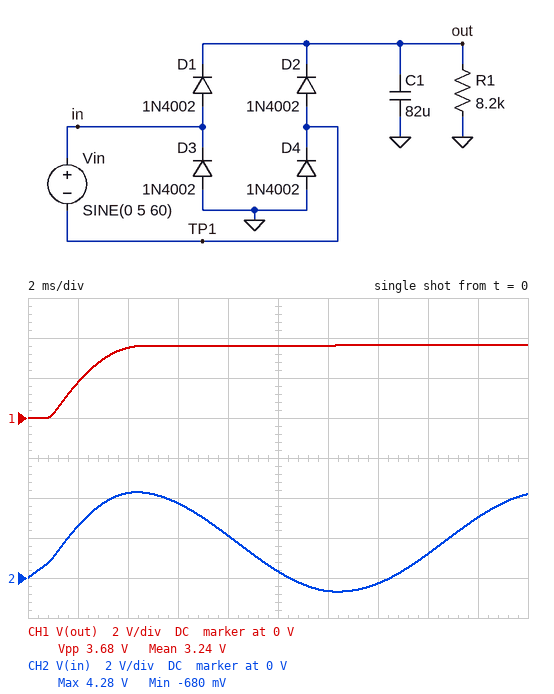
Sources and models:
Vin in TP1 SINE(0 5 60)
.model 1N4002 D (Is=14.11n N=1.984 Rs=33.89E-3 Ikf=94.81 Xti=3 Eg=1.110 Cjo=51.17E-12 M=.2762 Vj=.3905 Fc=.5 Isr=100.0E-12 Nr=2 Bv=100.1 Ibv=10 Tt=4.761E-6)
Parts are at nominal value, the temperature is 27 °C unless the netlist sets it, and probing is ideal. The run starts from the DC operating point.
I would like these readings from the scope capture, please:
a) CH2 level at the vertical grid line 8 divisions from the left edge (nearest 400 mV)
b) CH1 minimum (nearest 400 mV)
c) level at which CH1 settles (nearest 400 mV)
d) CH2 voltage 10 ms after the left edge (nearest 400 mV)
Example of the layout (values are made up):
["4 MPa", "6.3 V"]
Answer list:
["1.2 V", "0 V", "3.6 V", "400 mV"]
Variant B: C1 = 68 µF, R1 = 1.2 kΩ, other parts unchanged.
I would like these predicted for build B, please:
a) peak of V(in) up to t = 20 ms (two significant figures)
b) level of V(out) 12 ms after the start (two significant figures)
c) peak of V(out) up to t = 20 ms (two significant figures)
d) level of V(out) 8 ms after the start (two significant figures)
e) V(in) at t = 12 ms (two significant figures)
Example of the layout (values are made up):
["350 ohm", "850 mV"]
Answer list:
["4.3 V", "3.4 V", "3.6 V", "3.5 V", "-740 mV"]
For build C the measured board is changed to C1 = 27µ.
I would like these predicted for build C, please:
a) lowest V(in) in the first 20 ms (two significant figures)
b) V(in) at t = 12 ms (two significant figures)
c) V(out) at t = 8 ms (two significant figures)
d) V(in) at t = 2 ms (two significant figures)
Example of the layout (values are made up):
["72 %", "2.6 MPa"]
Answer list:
["-650 mV", "-630 mV", "3.7 V", "2.7 V"]
